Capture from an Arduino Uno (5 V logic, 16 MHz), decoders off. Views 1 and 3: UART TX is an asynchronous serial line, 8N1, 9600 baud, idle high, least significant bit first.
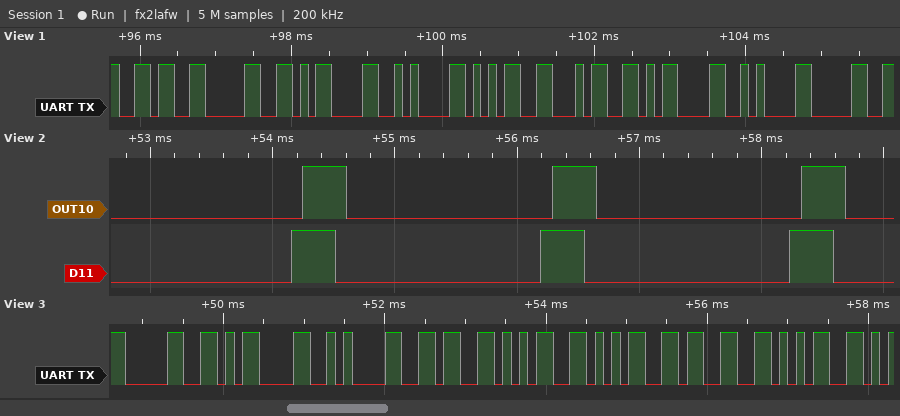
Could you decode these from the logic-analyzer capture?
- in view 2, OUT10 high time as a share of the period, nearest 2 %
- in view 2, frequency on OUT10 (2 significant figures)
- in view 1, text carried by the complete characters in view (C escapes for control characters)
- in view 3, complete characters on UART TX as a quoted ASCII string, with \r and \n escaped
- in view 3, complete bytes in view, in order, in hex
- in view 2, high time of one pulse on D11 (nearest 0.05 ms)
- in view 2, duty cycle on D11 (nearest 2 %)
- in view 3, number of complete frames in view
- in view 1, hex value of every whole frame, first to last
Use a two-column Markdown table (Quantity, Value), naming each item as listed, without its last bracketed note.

| Quantity | Value |
|---|---|
| in view 2, OUT10 high time as a share of the period, nearest 2 % | 18 % |
| in view 2, frequency on OUT10 | 490 Hz |
| in view 1, text carried by the complete characters in view | "60\r\n54\r\n0" |
| in view 3, complete characters on UART TX as a quoted ASCII string, with \r and \n escaped | "0\r\n65535" |
| in view 3, complete bytes in view, in order, in hex | 30 0D 0A 36 35 35 33 35 |
| in view 2, high time of one pulse on D11 | 0.35 ms |
| in view 2, duty cycle on D11 | 18 % |
| in view 3, number of complete frames in view | 8 |
| in view 1, hex value of every whole frame, first to last | 36 30 0D 0A 35 34 0D 0A 30 |
